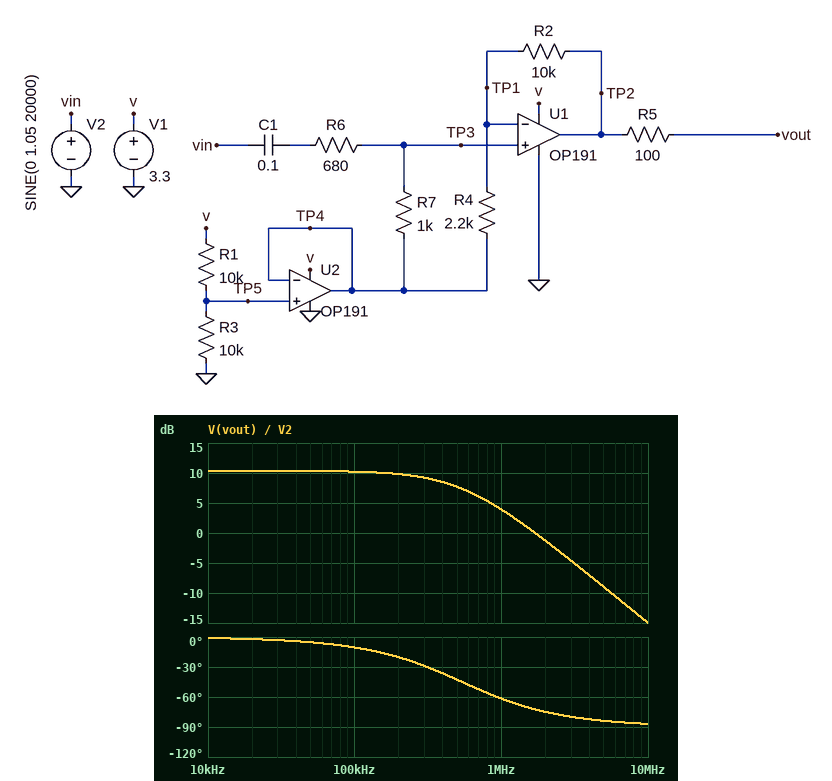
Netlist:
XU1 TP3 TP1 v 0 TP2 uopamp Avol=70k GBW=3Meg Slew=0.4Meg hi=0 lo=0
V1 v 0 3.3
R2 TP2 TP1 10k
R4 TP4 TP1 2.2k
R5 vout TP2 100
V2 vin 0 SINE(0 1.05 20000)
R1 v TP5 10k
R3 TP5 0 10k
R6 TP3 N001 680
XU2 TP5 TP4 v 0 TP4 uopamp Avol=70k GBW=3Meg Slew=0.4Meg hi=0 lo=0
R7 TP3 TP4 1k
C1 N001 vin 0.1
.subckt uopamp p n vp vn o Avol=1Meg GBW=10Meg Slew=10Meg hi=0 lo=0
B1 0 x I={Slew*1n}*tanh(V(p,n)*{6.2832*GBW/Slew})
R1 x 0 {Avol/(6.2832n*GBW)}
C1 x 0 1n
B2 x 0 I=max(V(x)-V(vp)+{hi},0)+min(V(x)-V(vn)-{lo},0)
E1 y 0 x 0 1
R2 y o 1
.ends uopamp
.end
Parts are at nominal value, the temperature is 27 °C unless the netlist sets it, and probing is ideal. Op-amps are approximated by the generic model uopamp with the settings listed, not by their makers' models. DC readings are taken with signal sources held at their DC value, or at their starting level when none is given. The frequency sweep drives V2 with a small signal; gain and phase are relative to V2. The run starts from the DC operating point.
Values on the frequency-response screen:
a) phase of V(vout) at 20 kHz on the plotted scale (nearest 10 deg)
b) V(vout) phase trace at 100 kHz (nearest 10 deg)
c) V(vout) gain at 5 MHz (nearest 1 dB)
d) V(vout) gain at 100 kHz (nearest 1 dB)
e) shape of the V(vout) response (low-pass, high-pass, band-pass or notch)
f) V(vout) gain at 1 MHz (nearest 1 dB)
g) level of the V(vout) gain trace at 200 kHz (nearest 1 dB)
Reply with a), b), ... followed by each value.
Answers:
a) 0 deg
b) -10 deg
c) -9 dB
d) 10 dB
e) low-pass
f) 4 dB
g) 10 dB
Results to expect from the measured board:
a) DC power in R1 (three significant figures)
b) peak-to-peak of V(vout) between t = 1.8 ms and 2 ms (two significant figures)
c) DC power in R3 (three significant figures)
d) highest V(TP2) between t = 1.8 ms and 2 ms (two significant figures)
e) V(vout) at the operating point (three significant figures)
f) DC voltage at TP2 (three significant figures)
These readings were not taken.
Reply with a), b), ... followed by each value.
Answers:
a) 272 µW
b) 3.3 V
c) 272 µW
d) 3.3 V
e) 1.65 V
f) 1.65 V
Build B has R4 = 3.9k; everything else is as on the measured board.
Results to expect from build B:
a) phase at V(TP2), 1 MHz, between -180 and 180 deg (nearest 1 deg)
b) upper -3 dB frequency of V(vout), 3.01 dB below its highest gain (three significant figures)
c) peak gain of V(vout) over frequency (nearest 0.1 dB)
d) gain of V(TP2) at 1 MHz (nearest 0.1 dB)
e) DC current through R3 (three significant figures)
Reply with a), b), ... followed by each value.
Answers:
a) -50 deg
b) 842 kHz
c) 6.5 dB
d) 2.7 dB
e) 165 µA
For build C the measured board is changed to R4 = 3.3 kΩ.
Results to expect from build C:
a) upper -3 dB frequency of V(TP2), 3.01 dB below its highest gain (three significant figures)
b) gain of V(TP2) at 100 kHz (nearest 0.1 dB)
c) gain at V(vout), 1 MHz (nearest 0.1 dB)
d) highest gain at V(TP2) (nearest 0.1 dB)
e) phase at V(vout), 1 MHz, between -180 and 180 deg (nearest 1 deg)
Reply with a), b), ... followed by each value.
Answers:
a) 744 kHz
b) 7.5 dB
c) 3.1 dB
d) 7.6 dB
e) -53 deg
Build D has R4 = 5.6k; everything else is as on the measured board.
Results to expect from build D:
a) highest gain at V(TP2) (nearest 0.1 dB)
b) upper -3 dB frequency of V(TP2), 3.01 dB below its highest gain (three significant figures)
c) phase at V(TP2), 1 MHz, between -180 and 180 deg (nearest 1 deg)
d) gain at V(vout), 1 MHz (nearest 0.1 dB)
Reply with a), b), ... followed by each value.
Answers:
a) 4.4 dB
b) 1.08 MHz
c) -43 deg
d) 1.7 dB
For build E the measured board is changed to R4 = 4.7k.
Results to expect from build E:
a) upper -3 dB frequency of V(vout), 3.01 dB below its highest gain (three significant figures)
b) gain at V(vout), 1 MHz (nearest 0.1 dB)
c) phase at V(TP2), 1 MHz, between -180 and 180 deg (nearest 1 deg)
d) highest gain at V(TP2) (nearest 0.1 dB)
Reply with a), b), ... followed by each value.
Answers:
a) 959 kHz
b) 2.2 dB
c) -46 deg
d) 5.4 dB
